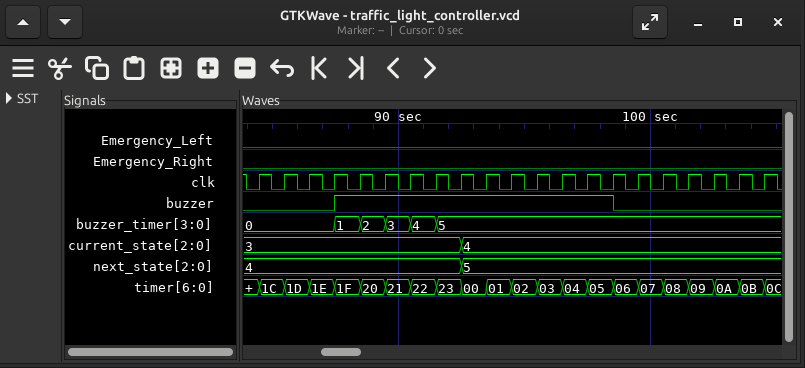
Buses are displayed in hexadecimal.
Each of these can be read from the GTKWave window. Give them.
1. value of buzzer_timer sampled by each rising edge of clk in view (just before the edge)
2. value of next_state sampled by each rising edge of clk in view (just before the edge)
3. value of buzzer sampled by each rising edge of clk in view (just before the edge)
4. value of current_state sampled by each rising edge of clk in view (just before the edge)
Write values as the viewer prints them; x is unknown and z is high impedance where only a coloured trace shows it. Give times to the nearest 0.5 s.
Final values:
0, 0, 0, 0, 1, 2, 3, 4, 5, 5, 5, 5, 5, 5, 5, 5, 5, 5, 5, 5, 5
4, 4, 4, 4, 4, 4, 4, 4, 4, 5, 5, 5, 5, 5, 5, 5, 5, 5, 5, 5, 5
0 0 0 0 1 1 1 1 1 1 1 1 1 1 1 0 0 0 0 0 0
3, 3, 3, 3, 3, 3, 3, 3, 3, 4, 4, 4, 4, 4, 4, 4, 4, 4, 4, 4, 4
